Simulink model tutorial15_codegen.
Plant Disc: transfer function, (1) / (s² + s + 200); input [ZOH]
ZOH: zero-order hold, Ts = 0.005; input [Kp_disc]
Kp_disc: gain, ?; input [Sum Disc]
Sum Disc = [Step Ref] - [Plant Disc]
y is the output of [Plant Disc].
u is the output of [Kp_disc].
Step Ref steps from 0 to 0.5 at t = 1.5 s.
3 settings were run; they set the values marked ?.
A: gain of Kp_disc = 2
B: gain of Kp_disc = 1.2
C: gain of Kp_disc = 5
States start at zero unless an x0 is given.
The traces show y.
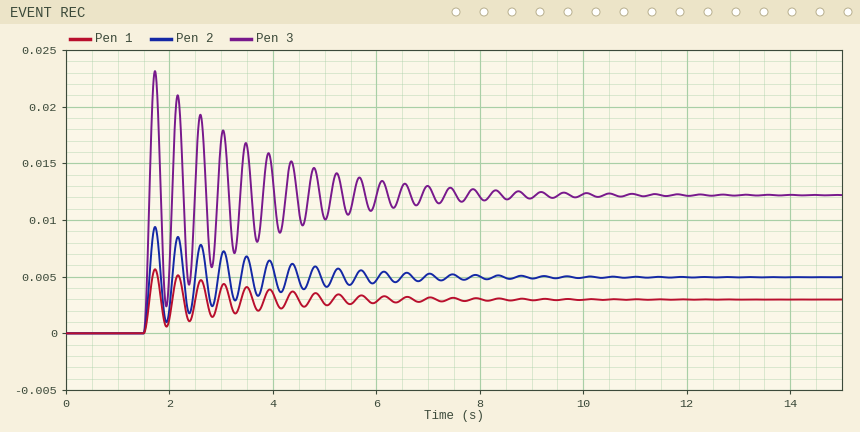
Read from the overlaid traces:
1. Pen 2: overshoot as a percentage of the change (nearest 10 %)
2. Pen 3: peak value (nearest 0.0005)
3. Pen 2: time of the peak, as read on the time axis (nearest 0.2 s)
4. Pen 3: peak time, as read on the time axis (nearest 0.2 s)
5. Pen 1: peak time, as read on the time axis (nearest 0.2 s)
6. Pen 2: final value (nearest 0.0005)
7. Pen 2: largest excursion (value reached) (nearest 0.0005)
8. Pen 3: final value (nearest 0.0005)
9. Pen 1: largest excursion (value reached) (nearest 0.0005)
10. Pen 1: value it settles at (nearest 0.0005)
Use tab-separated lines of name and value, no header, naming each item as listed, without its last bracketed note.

Pen 2: overshoot as a percentage of the change	90 %
Pen 3: peak value	0.0230
Pen 2: time of the peak, as read on the time axis	1.8 s
Pen 3: peak time, as read on the time axis	1.8 s
Pen 1: peak time, as read on the time axis	1.8 s
Pen 2: final value	0.0050
Pen 2: largest excursion (value reached)	0.0095
Pen 3: final value	0.0120
Pen 1: largest excursion (value reached)	0.0055
Pen 1: value it settles at	0.0030
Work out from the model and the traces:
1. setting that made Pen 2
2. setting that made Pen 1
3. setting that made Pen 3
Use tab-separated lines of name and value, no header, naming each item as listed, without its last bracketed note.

setting that made Pen 2	A
setting that made Pen 1	B
setting that made Pen 3	C
